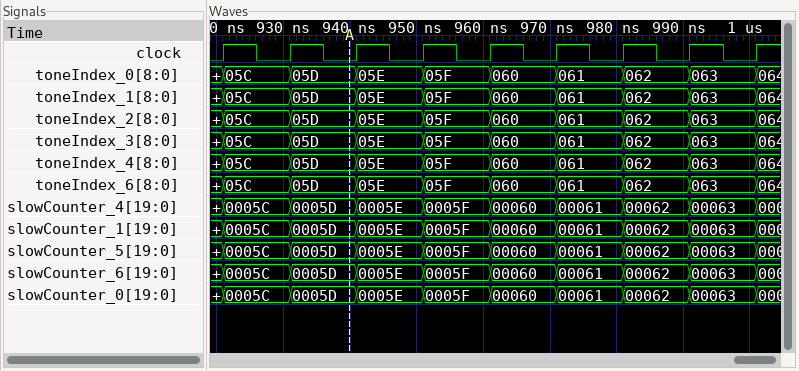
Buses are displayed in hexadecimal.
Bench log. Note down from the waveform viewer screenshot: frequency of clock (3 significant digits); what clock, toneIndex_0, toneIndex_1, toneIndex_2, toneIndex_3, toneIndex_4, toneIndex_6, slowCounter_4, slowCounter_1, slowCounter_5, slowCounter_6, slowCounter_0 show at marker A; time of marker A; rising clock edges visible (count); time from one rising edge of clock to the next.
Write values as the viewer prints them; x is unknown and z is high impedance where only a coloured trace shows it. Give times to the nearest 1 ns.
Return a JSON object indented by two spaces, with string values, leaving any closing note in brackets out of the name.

{
  "frequency of clock": "100 MHz",
  "what clock, toneIndex_0, toneIndex_1, toneIndex_2, toneIndex_3, toneIndex_4, toneIndex_6, slowCounter_4, slowCounter_1, slowCounter_5, slowCounter_6, slowCounter_0 show at marker A": "clock=0, toneIndex_0=05D, toneIndex_1=05D, toneIndex_2=05D, toneIndex_3=05D, toneIndex_4=05D, toneIndex_6=05D, slowCounter_4=0005D, slowCounter_1=0005D, slowCounter_5=0005D, slowCounter_6=0005D, slowCounter_0=0005D",
  "time of marker A": "940 ns",
  "rising clock edges visible": "9",
  "time from one rising edge of clock to the next": "10 ns"
}
